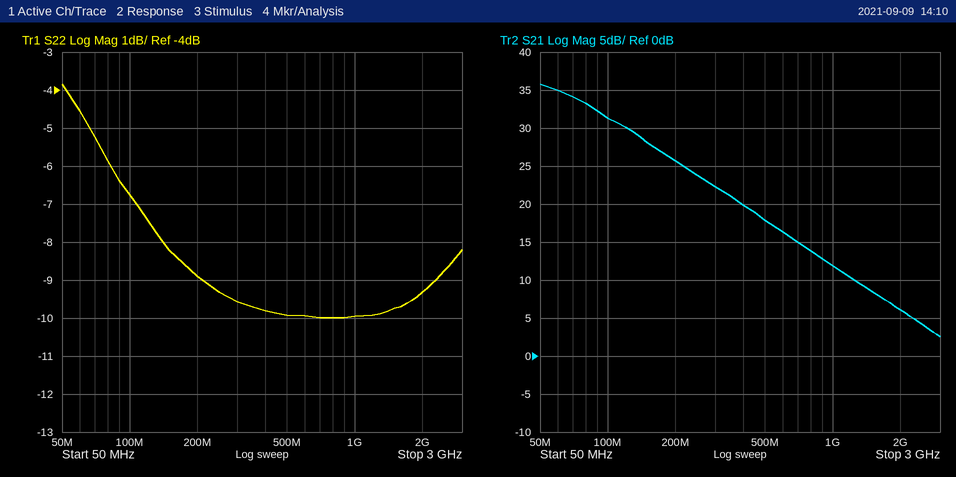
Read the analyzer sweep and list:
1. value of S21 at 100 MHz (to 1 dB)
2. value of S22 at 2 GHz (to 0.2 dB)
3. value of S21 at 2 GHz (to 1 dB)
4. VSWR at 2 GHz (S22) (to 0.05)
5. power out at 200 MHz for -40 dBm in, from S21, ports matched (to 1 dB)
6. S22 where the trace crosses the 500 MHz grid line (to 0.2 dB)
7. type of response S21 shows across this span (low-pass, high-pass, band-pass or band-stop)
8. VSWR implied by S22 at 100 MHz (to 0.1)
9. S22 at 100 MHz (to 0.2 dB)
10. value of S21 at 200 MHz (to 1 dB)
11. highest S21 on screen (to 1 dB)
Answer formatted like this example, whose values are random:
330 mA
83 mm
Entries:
31 dB
-9.4 dB
6 dB
2.05
-14 dBm
-10.0 dB
low-pass
2.7
-6.8 dB
26 dB
36 dB
